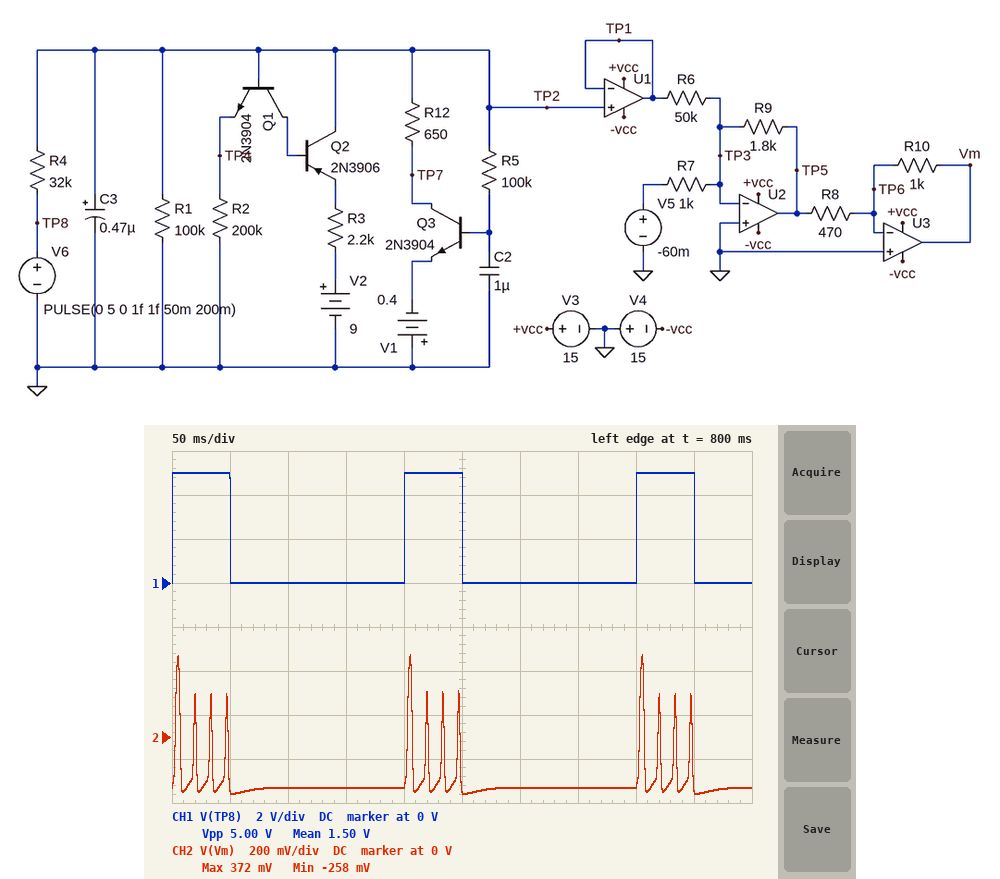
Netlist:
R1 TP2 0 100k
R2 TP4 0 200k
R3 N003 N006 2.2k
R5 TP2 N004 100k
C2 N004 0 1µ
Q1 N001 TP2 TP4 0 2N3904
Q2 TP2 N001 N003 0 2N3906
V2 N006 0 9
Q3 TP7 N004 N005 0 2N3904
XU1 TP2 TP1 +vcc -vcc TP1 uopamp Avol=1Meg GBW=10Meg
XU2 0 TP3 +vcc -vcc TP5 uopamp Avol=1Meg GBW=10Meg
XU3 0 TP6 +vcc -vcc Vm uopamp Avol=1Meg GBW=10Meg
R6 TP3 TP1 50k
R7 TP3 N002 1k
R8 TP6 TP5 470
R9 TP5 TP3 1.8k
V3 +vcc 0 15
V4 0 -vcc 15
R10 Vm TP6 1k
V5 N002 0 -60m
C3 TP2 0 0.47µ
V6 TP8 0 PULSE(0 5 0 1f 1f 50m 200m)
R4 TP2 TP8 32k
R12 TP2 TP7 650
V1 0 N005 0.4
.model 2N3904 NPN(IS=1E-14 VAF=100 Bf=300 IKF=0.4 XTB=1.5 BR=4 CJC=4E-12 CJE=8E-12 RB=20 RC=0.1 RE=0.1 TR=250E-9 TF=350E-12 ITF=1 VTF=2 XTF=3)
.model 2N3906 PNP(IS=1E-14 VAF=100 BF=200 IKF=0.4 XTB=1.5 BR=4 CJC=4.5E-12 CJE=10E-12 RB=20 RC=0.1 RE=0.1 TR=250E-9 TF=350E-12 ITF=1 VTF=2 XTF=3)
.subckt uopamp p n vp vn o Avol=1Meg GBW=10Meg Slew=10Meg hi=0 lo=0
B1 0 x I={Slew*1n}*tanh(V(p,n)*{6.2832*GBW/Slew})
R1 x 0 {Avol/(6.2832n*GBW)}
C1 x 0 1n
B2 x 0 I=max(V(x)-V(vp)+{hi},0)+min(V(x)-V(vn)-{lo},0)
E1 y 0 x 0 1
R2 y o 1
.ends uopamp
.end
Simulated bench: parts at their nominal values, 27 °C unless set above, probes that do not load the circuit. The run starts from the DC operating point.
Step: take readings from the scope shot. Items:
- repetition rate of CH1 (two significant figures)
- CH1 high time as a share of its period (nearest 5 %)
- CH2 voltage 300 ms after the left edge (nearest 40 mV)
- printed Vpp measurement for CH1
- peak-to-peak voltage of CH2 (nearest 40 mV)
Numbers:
5.0 Hz
25 %
-240 mV
5.00 V
640 mV
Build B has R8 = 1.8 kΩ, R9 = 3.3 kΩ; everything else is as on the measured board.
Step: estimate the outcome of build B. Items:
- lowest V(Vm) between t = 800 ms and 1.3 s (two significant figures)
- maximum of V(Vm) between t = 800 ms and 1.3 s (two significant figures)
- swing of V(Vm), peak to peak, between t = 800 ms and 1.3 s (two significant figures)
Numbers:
-120 mV
180 mV
300 mV
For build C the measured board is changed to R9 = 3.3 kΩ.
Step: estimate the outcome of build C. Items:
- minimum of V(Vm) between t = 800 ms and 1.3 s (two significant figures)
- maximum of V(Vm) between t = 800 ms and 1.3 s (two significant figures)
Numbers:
-470 mV
680 mV
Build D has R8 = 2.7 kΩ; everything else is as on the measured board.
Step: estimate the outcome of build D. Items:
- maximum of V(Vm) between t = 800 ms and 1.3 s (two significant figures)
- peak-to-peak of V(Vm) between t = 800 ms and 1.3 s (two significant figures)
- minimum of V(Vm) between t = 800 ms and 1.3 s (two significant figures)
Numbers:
65 mV
110 mV
-45 mV
